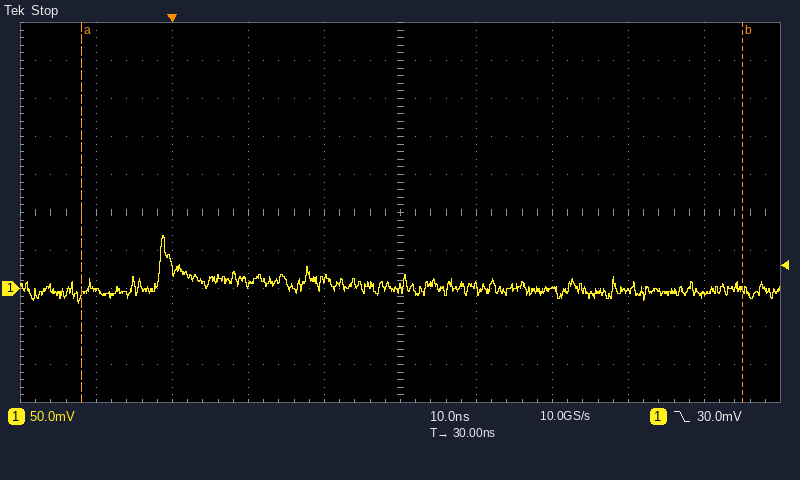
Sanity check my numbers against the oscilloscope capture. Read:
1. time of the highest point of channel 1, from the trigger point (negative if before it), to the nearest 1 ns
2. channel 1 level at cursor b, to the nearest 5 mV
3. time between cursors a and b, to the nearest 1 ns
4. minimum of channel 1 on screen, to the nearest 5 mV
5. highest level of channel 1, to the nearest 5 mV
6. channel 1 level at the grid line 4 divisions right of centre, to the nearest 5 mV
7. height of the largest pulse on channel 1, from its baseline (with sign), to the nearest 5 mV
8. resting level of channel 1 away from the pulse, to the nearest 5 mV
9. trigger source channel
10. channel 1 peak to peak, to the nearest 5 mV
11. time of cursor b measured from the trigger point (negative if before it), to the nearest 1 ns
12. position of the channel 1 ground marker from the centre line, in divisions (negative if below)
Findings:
-1 ns
0 mV
87 ns
-20 mV
70 mV
-10 mV
+70 mV
0 mV
channel 1
90 mV
+75 ns
-2.0 div
